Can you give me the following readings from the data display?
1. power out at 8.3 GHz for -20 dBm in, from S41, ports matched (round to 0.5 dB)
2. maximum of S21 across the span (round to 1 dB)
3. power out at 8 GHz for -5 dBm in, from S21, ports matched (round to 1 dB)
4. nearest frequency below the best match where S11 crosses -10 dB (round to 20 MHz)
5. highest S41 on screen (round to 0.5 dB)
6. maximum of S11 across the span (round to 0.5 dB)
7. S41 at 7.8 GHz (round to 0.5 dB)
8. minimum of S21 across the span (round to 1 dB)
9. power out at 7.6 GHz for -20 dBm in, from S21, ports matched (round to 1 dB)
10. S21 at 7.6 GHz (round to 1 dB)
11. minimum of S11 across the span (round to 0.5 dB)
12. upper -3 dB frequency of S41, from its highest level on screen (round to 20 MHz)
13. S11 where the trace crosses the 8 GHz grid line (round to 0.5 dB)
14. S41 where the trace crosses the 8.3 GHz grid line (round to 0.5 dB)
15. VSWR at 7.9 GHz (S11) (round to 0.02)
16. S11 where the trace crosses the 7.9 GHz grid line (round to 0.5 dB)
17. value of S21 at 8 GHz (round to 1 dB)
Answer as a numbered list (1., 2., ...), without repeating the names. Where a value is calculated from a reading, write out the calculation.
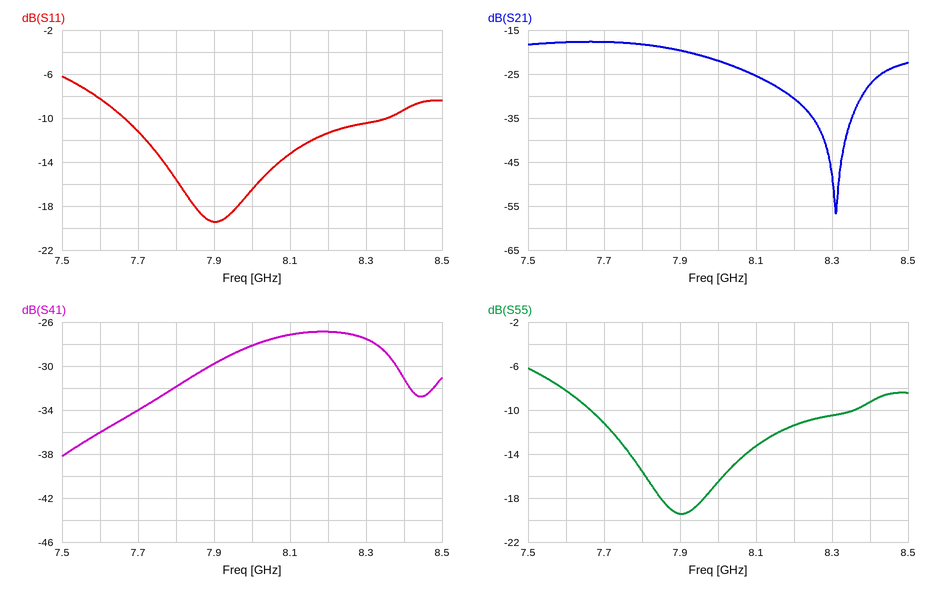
1. -20 dBm + (-27.5 dB) = -47.5 dBm
2. -18 dB
3. -5 dBm + (-22 dB) = -27 dBm
4. 7.66 GHz
5. -27.0 dB
6. -6.0 dB
7. -32.0 dB
8. -57 dB
9. -20 dBm + (-18 dB) = -38 dBm
10. -18 dB
11. -19.5 dB
12. 8.38 GHz
13. -16.5 dB
14. -27.5 dB
15. |Γ| = 10^(-19.5/20) = 0.1059; VSWR = (1 + 0.1059)/(1 − 0.1059) ≈ 1.24
16. -19.5 dB
17. -22 dB
